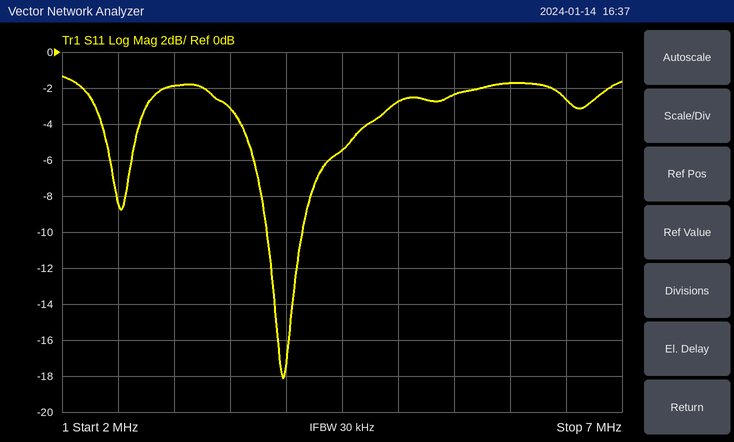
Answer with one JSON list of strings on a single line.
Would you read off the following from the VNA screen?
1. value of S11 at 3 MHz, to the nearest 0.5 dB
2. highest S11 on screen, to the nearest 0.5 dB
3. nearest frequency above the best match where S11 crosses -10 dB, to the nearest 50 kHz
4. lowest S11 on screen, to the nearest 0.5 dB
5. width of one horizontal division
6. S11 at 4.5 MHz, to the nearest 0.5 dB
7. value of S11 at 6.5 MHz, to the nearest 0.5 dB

["-2.0 dB", "-1.5 dB", "4.15 MHz", "-18.0 dB", "500 kHz", "-5.5 dB", "-2.5 dB"]
